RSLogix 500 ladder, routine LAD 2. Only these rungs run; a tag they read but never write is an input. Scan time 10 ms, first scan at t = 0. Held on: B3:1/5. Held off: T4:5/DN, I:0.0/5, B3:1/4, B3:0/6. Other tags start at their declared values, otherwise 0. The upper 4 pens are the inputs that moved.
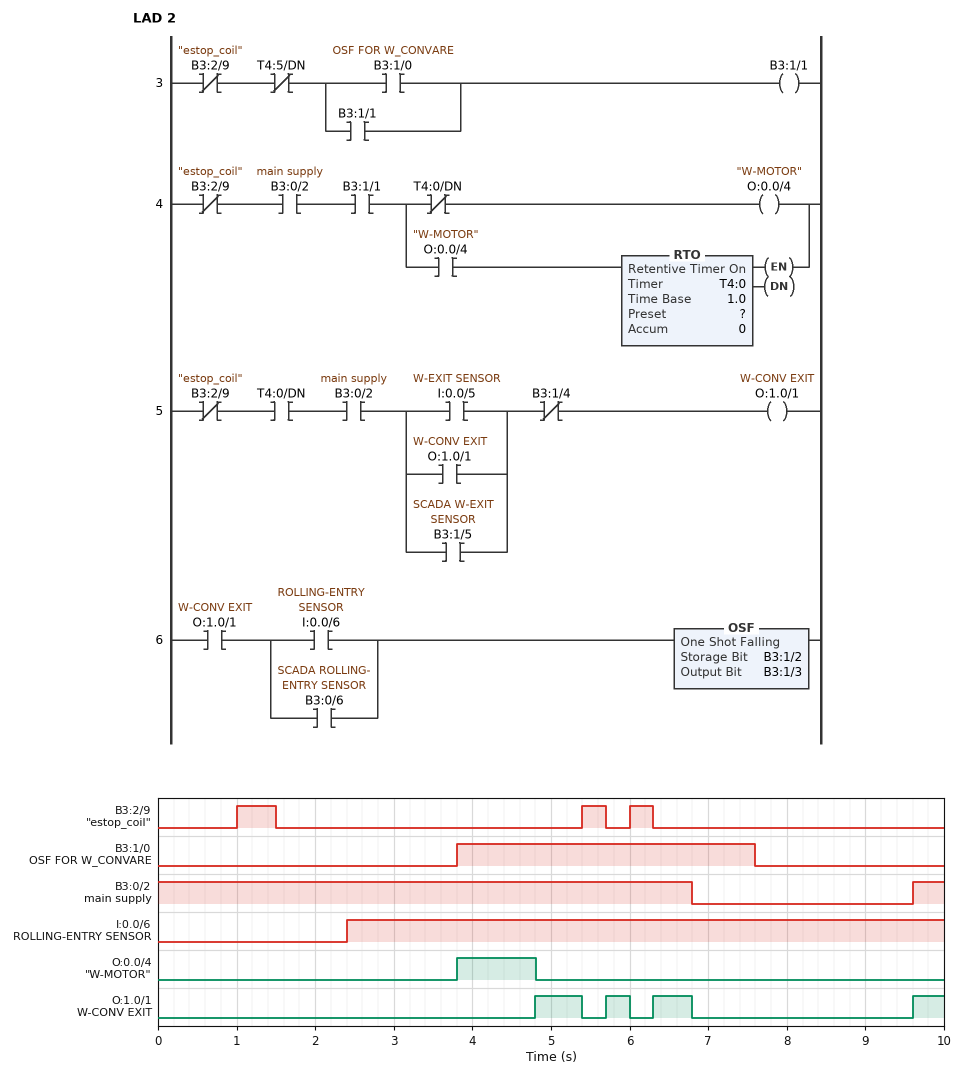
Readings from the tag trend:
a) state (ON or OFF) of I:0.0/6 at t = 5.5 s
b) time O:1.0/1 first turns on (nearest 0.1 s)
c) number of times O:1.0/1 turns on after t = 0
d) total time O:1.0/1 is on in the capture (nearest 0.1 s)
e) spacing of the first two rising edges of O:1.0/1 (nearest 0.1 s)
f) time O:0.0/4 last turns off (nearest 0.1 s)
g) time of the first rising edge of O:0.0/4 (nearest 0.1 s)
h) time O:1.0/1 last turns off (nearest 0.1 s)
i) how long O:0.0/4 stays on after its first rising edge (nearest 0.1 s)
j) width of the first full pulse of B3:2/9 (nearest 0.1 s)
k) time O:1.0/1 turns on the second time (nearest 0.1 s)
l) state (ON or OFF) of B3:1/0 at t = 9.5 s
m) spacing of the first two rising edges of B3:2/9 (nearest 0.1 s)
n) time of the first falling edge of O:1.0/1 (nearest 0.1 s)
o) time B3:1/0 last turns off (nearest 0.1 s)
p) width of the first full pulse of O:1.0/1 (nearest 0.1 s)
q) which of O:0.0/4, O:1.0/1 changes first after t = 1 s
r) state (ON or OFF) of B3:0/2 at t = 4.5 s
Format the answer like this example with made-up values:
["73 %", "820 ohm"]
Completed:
["ON", "4.8 s", "4", "1.8 s", "0.9 s", "4.8 s", "3.8 s", "6.8 s", "1.0 s", "0.5 s", "5.7 s", "OFF", "4.4 s", "5.4 s", "7.6 s", "0.6 s", "O:0.0/4", "ON"]
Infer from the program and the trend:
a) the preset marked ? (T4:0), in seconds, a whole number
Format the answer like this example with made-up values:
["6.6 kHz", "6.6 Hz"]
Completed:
["1 s"]
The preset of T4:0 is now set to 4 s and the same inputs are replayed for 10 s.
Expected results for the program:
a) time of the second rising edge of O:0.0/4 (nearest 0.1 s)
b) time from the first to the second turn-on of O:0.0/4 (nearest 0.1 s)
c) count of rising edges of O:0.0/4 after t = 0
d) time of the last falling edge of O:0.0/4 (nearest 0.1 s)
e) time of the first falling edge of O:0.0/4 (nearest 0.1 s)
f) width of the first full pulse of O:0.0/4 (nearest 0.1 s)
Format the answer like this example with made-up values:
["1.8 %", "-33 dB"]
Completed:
["5.7 s", "1.9 s", "4", "6.8 s", "5.4 s", "1.6 s"]
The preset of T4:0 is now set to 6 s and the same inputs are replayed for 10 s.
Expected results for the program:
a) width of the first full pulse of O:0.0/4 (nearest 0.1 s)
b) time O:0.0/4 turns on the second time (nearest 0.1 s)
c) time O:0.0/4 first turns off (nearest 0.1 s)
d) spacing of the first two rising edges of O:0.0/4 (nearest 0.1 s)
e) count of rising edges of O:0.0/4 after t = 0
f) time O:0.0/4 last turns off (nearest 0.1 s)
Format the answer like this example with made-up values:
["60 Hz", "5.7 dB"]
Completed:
["1.6 s", "5.7 s", "5.4 s", "1.9 s", "4", "6.8 s"]
